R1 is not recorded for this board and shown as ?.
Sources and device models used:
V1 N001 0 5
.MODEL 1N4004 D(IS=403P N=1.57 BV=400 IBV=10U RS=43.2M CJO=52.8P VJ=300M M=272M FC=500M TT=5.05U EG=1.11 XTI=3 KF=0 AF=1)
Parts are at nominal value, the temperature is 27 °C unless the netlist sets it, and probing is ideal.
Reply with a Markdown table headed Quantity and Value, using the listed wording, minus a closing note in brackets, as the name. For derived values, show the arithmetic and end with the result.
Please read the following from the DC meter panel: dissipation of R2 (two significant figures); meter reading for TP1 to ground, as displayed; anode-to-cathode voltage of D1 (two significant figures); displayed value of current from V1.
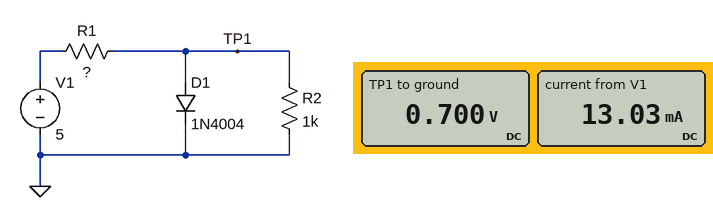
| Quantity | Value |
|---|---|
| dissipation of R2 | (700 mV)^2 / 1 kΩ = 490 µW |
| meter reading for TP1 to ground, as displayed | 0.700 V |
| anode-to-cathode voltage of D1 | 700 mV = 700 mV |
| displayed value of current from V1 | 13.03 mA |
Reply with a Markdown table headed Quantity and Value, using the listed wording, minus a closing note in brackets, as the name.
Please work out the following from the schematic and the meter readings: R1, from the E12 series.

| Quantity | Value |
|---|---|
| R1, from the E12 series | 330 Ω |
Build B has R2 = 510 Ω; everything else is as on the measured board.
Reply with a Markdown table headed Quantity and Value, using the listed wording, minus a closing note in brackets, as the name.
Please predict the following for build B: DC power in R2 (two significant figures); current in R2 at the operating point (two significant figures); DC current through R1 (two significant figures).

| Quantity | Value |
|---|---|
| DC power in R2 | 960 µW |
| current in R2 at the operating point | 1.4 mA |
| DC current through R1 | 13 mA |
